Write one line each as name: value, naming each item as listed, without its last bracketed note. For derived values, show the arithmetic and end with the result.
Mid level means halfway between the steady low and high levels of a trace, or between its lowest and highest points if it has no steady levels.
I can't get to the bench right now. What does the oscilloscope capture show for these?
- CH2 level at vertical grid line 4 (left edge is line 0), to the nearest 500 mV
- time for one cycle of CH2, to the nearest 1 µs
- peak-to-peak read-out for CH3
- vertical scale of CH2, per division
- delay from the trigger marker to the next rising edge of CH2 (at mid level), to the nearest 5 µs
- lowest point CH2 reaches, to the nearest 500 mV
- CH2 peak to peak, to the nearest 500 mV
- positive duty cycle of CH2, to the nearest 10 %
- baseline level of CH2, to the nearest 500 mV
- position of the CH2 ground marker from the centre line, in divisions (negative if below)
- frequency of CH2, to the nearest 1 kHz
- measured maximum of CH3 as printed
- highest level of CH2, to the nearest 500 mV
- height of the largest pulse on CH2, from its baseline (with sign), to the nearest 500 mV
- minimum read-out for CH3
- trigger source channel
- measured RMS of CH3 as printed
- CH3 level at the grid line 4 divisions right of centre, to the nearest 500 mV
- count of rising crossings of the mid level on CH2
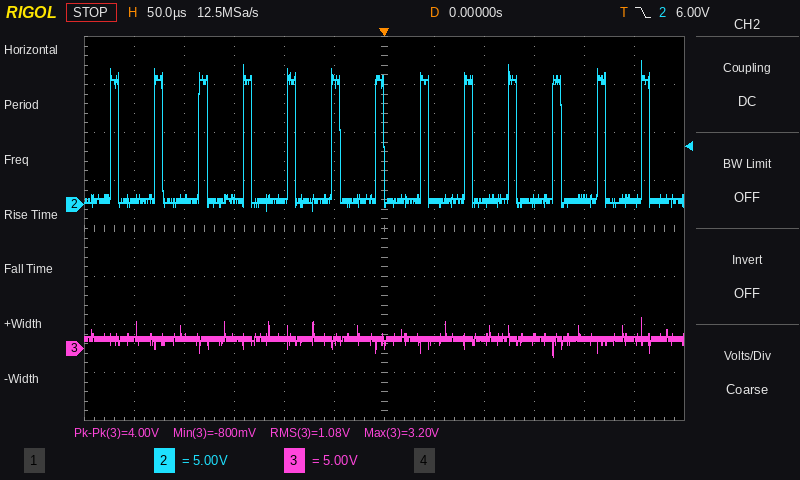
CH2 level at vertical grid line 4 (left edge is line 0), to the nearest 500 mV: 500 mV
time for one cycle of CH2, to the nearest 1 µs: 44 µs
peak-to-peak read-out for CH3: 4.00 V
vertical scale of CH2, per division: 5 V
delay from the trigger marker to the next rising edge of CH2 (at mid level), to the nearest 5 µs: 35 µs
lowest point CH2 reaches, to the nearest 500 mV: -500 mV
CH2 peak to peak, to the nearest 500 mV: 15.0 V − (-500 mV) = 15.5 V
positive duty cycle of CH2, to the nearest 10 %: 20 %
baseline level of CH2, to the nearest 500 mV: 500 mV
position of the CH2 ground marker from the centre line, in divisions: +0.5 div
frequency of CH2, to the nearest 1 kHz: 1 / 44 µs ≈ 23 kHz
measured maximum of CH3 as printed: 3.20 V
highest level of CH2, to the nearest 500 mV: 15.0 V
height of the largest pulse on CH2, from its baseline (with sign), to the nearest 500 mV: 15.0 V − (500 mV) = +14.5 V
minimum read-out for CH3: -800 mV
trigger source channel: CH2
measured RMS of CH3 as printed: 1.08 V
CH3 level at the grid line 4 divisions right of centre, to the nearest 500 mV: 1.0 V
count of rising crossings of the mid level on CH2: 13
